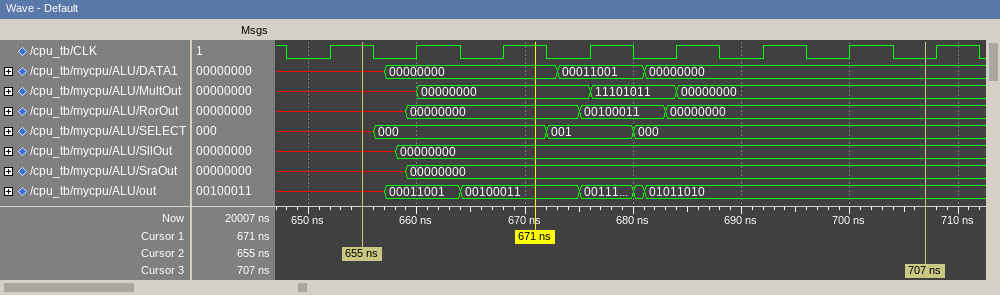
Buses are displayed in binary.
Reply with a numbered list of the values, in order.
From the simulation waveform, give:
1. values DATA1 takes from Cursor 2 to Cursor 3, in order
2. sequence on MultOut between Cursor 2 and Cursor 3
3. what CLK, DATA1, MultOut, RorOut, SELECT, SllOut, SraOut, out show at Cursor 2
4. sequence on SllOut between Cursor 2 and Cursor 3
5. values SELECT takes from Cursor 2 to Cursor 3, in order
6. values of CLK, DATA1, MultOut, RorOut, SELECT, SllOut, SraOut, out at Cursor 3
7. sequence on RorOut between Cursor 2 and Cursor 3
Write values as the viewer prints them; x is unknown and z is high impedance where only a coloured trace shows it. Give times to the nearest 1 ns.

1. x, 00000000, 00011001, 00000000
2. x, 00000000, 11101011, 00000000
3. CLK=1, DATA1=x, MultOut=x, RorOut=x, SELECT=x, SllOut=x, SraOut=x, out=x
4. x, 00000000
5. x, 000, 001, 000
6. CLK=0, DATA1=00000000, MultOut=00000000, RorOut=00000000, SELECT=000, SllOut=00000000, SraOut=00000000, out=01011010
7. x, 00000000, 00100011, 00000000
